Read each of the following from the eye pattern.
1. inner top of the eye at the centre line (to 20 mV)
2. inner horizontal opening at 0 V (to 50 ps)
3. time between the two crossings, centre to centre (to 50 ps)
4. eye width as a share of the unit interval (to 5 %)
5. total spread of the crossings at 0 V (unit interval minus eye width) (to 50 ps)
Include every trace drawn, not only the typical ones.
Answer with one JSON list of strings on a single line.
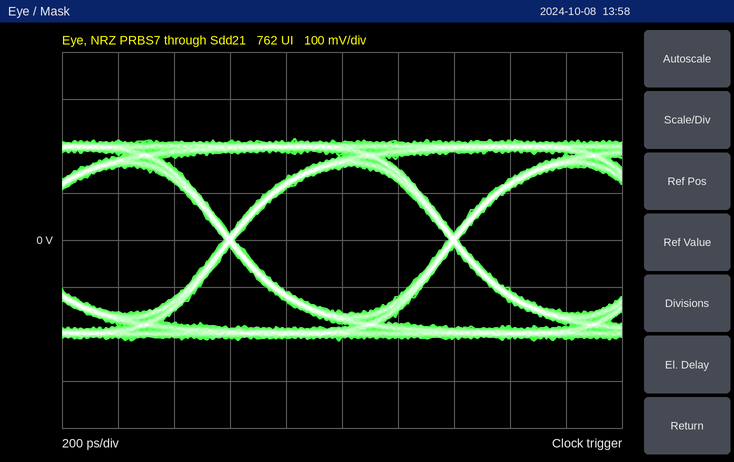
["160 mV", "750 ps", "800 ps", "95 %", "50 ps"]
